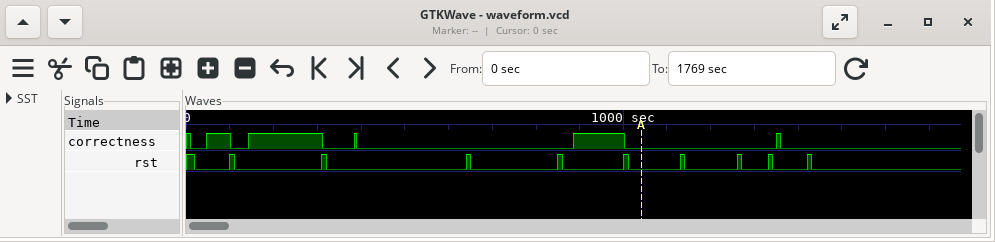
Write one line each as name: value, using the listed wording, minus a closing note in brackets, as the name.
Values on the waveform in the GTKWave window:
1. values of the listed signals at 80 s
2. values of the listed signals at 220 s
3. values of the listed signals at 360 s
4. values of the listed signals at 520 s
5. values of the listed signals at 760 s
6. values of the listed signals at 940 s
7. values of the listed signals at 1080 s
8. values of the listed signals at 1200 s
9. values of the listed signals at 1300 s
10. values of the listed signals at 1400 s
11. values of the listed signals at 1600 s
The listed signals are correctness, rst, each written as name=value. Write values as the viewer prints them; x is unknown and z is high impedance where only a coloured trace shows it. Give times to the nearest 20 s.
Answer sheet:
values of the listed signals at 80 s: correctness=1, rst=0
values of the listed signals at 220 s: correctness=1, rst=0
values of the listed signals at 360 s: correctness=0, rst=0
values of the listed signals at 520 s: correctness=0, rst=0
values of the listed signals at 760 s: correctness=0, rst=0
values of the listed signals at 940 s: correctness=1, rst=0
values of the listed signals at 1080 s: correctness=0, rst=0
values of the listed signals at 1200 s: correctness=0, rst=0
values of the listed signals at 1300 s: correctness=0, rst=0
values of the listed signals at 1400 s: correctness=0, rst=0
values of the listed signals at 1600 s: correctness=0, rst=0
